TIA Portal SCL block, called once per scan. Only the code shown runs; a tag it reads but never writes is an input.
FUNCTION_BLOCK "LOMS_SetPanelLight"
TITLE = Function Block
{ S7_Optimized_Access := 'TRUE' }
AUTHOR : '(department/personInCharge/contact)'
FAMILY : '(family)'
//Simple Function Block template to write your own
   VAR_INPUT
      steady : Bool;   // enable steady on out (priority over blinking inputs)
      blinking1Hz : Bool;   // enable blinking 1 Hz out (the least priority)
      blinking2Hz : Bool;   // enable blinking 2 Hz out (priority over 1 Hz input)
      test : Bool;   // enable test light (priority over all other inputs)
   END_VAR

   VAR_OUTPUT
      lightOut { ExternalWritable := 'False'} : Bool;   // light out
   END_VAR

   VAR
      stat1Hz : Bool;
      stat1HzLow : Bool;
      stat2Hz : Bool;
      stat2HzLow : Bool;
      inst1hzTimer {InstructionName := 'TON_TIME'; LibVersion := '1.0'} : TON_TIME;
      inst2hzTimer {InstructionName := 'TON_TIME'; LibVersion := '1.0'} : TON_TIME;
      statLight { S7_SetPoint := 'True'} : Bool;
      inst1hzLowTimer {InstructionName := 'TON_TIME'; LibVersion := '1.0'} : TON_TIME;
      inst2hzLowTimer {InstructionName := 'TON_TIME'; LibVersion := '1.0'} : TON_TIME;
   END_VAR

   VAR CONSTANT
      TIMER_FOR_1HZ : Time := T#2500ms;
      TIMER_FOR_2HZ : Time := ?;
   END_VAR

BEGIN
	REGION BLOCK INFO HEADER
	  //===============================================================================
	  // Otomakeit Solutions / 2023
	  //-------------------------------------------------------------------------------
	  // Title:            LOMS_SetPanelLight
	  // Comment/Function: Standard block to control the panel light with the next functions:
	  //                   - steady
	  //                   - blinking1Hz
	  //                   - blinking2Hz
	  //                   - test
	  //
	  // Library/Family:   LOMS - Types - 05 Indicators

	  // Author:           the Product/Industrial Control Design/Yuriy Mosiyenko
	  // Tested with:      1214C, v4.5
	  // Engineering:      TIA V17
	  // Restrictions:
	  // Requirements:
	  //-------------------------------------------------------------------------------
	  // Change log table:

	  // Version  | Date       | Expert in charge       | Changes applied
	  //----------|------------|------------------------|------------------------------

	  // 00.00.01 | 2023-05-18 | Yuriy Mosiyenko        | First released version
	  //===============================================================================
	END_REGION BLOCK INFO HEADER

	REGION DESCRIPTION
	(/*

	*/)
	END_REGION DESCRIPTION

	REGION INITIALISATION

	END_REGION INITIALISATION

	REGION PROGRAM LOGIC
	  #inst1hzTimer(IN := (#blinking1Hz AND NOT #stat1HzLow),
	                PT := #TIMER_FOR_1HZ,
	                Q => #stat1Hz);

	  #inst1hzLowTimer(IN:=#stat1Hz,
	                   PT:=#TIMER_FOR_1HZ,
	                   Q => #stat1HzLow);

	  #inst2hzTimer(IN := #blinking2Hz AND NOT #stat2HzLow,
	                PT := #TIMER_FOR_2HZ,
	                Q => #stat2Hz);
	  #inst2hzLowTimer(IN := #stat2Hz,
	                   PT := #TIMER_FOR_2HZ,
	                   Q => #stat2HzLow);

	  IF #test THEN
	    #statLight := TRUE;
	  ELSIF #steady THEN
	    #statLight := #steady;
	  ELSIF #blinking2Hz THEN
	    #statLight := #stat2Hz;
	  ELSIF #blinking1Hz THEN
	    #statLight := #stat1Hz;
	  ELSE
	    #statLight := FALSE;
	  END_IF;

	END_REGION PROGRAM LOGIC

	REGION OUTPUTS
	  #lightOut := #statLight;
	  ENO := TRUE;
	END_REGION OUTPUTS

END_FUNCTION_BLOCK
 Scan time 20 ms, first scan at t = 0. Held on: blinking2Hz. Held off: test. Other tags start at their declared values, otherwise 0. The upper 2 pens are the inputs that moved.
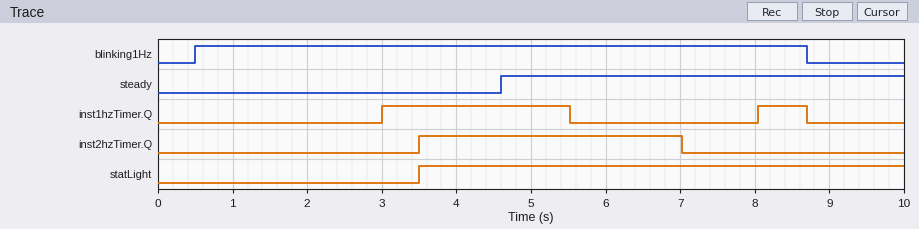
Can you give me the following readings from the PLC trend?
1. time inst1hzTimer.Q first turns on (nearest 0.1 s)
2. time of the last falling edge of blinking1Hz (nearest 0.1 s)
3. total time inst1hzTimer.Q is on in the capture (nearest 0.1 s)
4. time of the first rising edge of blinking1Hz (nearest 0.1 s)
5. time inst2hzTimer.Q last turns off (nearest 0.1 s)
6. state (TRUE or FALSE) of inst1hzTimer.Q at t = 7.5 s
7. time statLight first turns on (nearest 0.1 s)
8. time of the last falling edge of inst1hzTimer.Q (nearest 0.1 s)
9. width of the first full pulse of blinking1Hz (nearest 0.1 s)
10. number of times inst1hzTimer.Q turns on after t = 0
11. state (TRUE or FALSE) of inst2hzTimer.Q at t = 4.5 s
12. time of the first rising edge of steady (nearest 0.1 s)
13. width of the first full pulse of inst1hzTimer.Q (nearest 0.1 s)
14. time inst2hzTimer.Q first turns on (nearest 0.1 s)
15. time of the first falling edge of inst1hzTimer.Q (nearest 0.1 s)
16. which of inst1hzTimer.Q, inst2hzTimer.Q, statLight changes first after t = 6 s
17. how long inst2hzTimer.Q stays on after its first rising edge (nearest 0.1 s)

3.0 s
8.7 s
3.2 s
0.5 s
7.0 s
FALSE
3.5 s
8.7 s
8.2 s
2
TRUE
4.6 s
2.5 s
3.5 s
5.5 s
inst2hzTimer.Q
3.5 s
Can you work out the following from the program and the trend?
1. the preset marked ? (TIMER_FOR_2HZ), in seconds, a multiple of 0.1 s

3.5 s
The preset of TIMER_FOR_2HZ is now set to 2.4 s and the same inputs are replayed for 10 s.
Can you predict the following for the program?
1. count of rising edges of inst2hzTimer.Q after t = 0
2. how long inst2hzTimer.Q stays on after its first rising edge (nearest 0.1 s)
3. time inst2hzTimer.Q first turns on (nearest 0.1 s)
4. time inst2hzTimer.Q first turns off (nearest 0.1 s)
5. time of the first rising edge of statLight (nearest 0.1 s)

2
2.4 s
2.4 s
4.8 s
2.4 s
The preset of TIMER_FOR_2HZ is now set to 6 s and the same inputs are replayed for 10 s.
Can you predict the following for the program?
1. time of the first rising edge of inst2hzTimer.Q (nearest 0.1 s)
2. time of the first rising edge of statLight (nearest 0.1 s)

6.0 s
4.6 s
